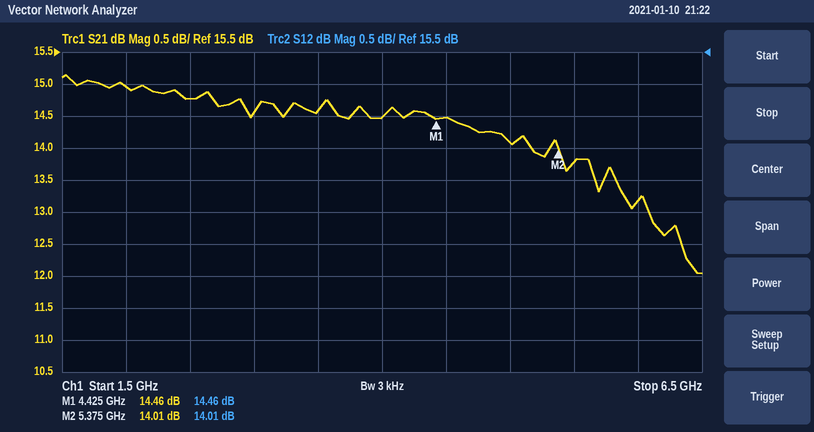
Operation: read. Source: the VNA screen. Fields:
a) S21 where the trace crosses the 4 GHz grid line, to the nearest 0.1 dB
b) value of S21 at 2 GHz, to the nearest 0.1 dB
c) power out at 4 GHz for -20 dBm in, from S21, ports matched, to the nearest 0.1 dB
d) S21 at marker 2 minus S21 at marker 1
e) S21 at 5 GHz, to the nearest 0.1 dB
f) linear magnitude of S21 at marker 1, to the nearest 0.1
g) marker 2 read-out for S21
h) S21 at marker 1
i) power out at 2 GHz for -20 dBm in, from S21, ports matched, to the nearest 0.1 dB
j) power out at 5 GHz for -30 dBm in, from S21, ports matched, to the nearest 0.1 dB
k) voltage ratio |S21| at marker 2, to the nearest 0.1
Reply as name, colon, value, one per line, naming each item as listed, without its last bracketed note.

S21 where the trace crosses the 4 GHz grid line, to the nearest 0.1 dB: 14.5 dB
value of S21 at 2 GHz, to the nearest 0.1 dB: 15.0 dB
power out at 4 GHz for -20 dBm in, from S21, ports matched, to the nearest 0.1 dB: -5.5 dBm
S21 at marker 2 minus S21 at marker 1: -0.45 dB
S21 at 5 GHz, to the nearest 0.1 dB: 14.1 dB
linear magnitude of S21 at marker 1, to the nearest 0.1: 5.3
marker 2 read-out for S21: 14.01 dB
S21 at marker 1: 14.46 dB
power out at 2 GHz for -20 dBm in, from S21, ports matched, to the nearest 0.1 dB: -5.0 dBm
power out at 5 GHz for -30 dBm in, from S21, ports matched, to the nearest 0.1 dB: -15.9 dBm
voltage ratio |S21| at marker 2, to the nearest 0.1: 5.0
